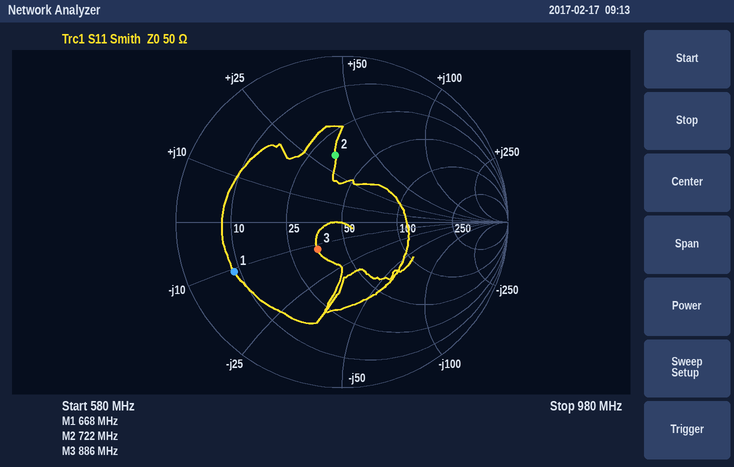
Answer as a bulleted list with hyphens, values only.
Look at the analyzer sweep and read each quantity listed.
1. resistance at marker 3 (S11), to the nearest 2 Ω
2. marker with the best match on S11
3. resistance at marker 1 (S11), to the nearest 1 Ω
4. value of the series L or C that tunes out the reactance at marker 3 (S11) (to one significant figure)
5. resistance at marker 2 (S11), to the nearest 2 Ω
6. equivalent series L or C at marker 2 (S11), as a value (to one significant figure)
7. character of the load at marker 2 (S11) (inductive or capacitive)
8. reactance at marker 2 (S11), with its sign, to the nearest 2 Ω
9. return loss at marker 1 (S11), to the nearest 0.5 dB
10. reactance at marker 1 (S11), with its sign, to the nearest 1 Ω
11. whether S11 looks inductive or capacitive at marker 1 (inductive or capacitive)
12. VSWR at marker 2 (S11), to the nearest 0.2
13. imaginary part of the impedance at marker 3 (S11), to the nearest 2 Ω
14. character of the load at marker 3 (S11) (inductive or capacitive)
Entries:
- 36 Ω
- marker 3
- 9 Ω
- 2 nH
- 34 Ω
- 7 nH
- inductive
- +32 Ω
- 3.0 dB
- -11 Ω
- capacitive
- 2.4
- -12 Ω
- capacitive
